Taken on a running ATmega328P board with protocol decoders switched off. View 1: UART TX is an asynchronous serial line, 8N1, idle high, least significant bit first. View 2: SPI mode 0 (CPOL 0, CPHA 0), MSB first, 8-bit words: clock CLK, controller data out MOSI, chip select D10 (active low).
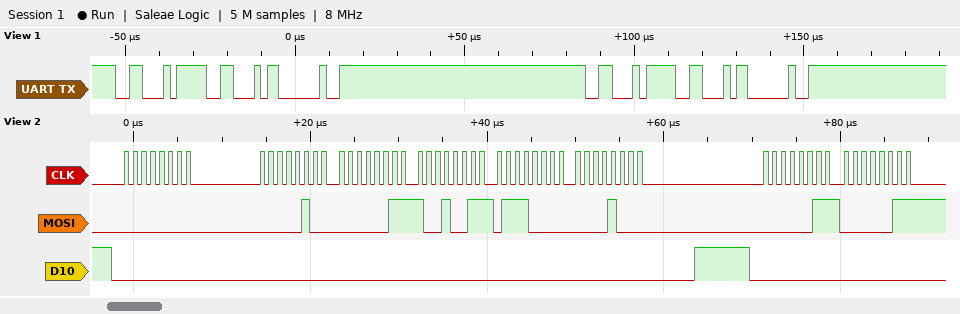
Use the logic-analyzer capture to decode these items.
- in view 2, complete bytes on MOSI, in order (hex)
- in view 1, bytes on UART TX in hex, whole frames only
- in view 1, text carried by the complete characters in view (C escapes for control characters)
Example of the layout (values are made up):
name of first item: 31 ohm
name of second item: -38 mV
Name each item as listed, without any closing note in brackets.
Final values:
in view 2, complete bytes on MOSI, in order: 00 04 03 93 70 08 03 03
in view 1, bytes on UART TX in hex, whole frames only: 46 46 20 46 46 20
in view 1, text carried by the complete characters in view: "FF FF "
